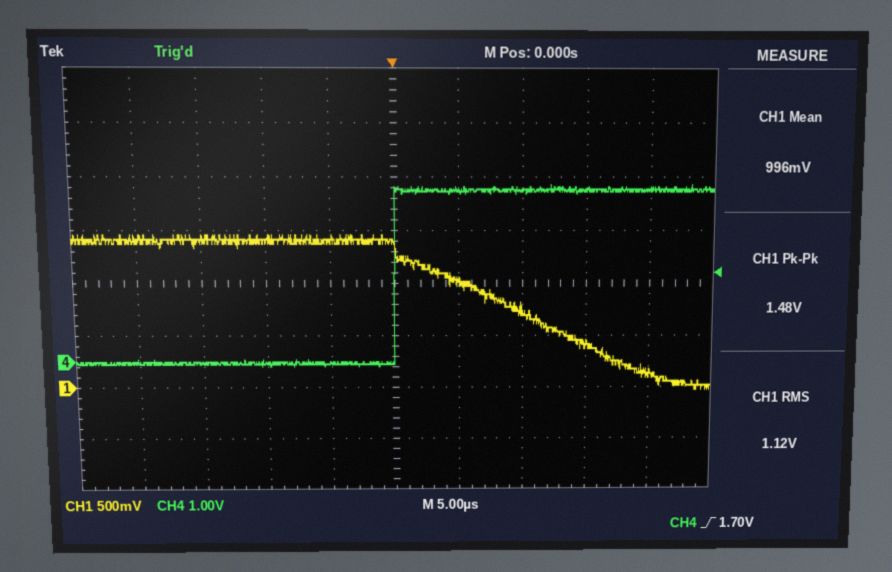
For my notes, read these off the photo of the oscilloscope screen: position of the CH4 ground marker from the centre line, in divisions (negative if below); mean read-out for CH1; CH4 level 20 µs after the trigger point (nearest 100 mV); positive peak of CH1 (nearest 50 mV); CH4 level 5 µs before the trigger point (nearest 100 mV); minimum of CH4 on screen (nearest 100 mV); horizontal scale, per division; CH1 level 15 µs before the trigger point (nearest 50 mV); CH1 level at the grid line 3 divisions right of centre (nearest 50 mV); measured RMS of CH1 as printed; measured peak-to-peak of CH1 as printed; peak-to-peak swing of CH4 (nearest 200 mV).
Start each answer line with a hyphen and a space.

- -1.5 div
- 996 mV
- 3.3 V
- 1.45 V
- 0.0 V
- -100 mV
- 5 µs
- 1.40 V
- 400 mV
- 1.12 V
- 1.48 V
- 3.4 V
